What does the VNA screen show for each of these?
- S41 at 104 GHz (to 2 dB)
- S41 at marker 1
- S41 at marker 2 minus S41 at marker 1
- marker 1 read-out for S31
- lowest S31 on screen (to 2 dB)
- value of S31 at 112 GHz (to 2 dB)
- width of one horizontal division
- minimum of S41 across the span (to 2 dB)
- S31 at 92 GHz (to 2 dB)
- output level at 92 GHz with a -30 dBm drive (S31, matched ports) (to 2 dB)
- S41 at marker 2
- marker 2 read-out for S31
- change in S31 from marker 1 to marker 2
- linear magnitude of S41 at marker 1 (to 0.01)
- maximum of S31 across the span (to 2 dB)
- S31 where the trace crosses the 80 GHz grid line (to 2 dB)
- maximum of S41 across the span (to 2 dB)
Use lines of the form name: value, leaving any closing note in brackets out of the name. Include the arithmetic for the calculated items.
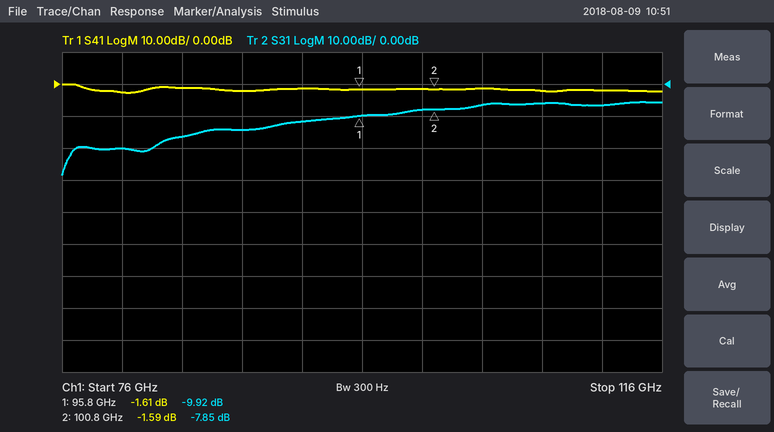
S41 at 104 GHz: -2 dB
S41 at marker 1: -1.61 dB
S41 at marker 2 minus S41 at marker 1: -1.59 − (-1.61) = 0.02 dB
marker 1 read-out for S31: -9.92 dB
lowest S31 on screen: -28 dB
value of S31 at 112 GHz: -6 dB
width of one horizontal division: 4 GHz
minimum of S41 across the span: -2 dB
S31 at 92 GHz: -12 dB
output level at 92 GHz with a -30 dBm drive (S31, matched ports): -30 dBm + (-12 dB) = -42 dBm
S41 at marker 2: -1.59 dB
marker 2 read-out for S31: -7.85 dB
change in S31 from marker 1 to marker 2: -7.85 − (-9.92) = 2.07 dB
linear magnitude of S41 at marker 1: 10^(-1.61/20) ≈ 0.83
maximum of S31 across the span: -6 dB
S31 where the trace crosses the 80 GHz grid line: -20 dB
maximum of S41 across the span: 0 dB
